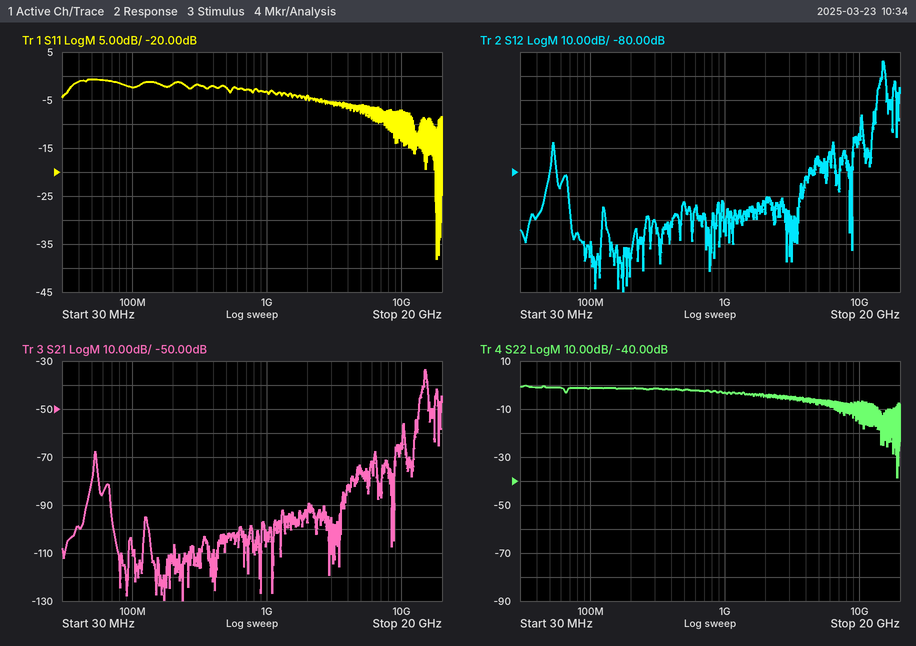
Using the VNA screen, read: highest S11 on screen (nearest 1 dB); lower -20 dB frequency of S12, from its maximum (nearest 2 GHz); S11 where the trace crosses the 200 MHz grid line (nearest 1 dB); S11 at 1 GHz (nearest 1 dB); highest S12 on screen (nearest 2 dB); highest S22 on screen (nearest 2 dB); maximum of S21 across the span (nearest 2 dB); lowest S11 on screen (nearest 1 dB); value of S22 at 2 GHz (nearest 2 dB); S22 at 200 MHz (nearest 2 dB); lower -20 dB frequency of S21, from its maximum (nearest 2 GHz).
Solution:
-1 dB
14 GHz
-2 dB
-3 dB
-34 dB
0 dB
-34 dB
-38 dB
-4 dB
-2 dB
14 GHz
